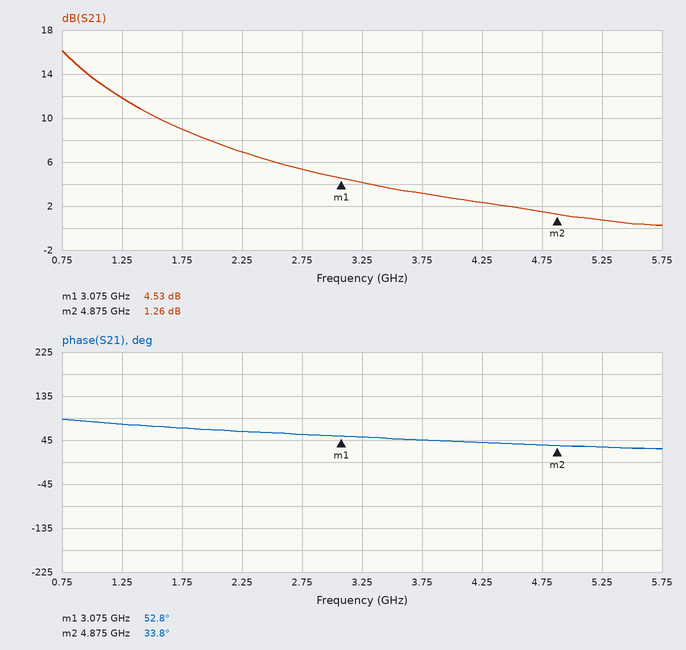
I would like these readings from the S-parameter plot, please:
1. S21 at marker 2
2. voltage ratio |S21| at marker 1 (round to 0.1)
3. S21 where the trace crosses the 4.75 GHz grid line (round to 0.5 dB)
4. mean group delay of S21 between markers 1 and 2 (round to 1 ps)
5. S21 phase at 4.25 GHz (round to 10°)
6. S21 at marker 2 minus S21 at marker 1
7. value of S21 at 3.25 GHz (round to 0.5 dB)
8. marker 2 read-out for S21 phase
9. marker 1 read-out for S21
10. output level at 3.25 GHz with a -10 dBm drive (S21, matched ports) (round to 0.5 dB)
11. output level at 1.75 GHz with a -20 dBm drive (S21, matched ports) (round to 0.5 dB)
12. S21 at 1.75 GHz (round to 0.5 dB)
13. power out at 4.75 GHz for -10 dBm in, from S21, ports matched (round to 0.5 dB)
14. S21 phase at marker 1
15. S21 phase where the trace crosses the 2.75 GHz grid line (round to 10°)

1.26 dB
1.7
1.5 dB
29 ps
40°
-3.27 dB
4.0 dB
33.8°
4.53 dB
-6.0 dBm
-11.0 dBm
9.0 dB
-8.5 dBm
52.8°
60°
